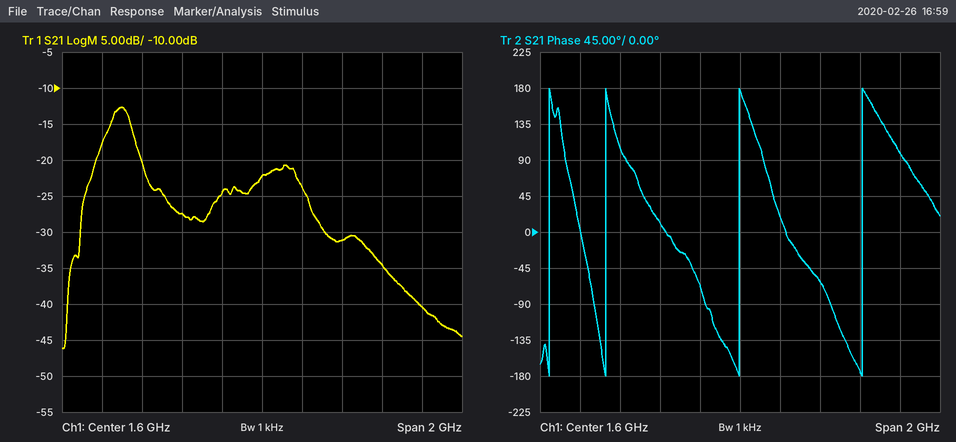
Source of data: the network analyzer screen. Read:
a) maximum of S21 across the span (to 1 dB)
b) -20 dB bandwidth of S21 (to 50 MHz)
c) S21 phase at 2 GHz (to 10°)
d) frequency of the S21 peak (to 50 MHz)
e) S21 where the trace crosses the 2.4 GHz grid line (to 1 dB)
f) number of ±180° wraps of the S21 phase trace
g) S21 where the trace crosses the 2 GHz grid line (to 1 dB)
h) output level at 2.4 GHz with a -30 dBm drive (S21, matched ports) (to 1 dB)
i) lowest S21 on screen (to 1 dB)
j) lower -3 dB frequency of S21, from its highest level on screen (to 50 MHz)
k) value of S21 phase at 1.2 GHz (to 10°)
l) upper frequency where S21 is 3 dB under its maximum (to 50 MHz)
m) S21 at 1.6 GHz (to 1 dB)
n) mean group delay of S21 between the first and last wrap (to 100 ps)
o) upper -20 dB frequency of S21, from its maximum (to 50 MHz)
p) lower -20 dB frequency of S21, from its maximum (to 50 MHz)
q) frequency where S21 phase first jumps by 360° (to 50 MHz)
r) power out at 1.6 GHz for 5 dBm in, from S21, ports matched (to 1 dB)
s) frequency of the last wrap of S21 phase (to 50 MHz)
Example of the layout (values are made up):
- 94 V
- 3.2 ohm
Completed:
- -13 dB
- 1.45 GHz
- -60°
- 900 MHz
- -40 dB
- 4
- -31 dB
- -70 dBm
- -46 dB
- 850 MHz
- 10°
- 950 MHz
- -22 dB
- 1.9 ns
- 2.15 GHz
- 700 MHz
- 650 MHz
- -17 dBm
- 2.20 GHz
